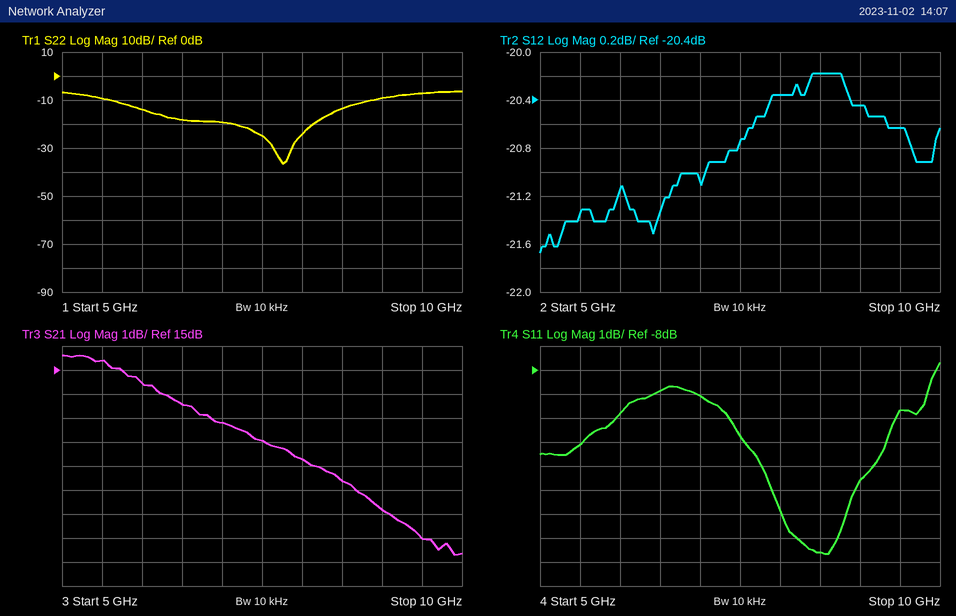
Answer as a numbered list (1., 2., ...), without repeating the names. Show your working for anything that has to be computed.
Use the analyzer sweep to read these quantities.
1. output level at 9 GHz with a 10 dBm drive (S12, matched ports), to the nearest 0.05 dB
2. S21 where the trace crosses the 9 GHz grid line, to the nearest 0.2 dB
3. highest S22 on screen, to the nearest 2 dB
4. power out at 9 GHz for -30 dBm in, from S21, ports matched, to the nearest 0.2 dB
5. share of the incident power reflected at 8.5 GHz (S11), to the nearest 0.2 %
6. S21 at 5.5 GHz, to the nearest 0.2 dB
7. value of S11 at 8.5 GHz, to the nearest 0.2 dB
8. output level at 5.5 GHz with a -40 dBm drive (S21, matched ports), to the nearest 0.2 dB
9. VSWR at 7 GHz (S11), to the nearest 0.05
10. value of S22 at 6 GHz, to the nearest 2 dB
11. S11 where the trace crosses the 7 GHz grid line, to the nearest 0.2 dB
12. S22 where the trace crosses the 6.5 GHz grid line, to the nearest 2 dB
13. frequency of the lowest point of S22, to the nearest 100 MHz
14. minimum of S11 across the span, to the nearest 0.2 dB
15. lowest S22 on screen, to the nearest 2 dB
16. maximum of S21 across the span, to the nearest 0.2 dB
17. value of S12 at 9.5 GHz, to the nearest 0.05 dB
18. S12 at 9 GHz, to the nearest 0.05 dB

1. 10 dBm + (-20.45 dB) = -10.45 dBm
2. 9.2 dB
3. -6 dB
4. -30 dBm + (9.2 dB) = -20.8 dBm
5. 10^(-15.6/10) ≈ 2.8 %
6. 15.4 dB
7. -15.6 dB
8. -40 dBm + (15.4 dB) = -24.6 dBm
9. |Γ| = 10^(-9/20) = 0.3548; VSWR = (1 + 0.3548)/(1 − 0.3548) ≈ 2.10
10. -14 dB
11. -9.0 dB
12. -18 dB
13. 7.8 GHz
14. -15.6 dB
15. -36 dB
16. 15.6 dB
17. -20.65 dB
18. -20.45 dB
